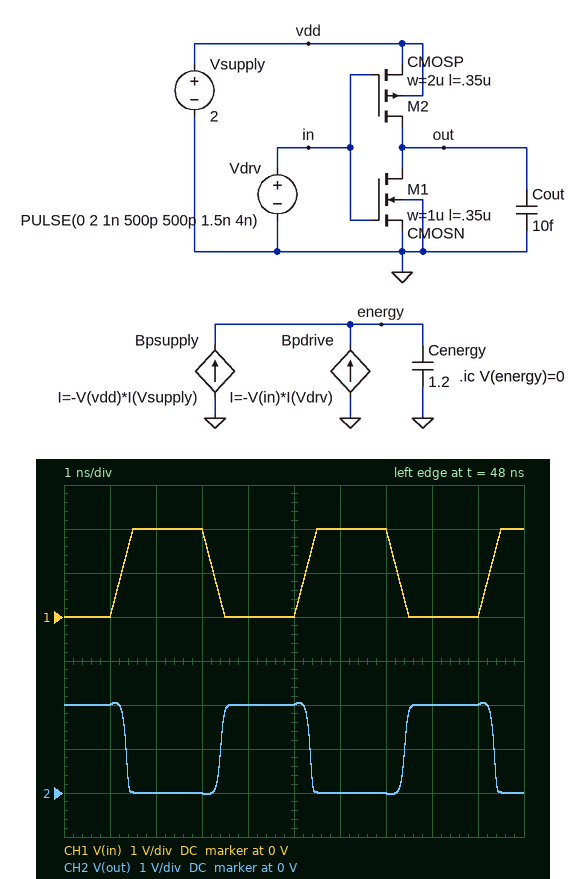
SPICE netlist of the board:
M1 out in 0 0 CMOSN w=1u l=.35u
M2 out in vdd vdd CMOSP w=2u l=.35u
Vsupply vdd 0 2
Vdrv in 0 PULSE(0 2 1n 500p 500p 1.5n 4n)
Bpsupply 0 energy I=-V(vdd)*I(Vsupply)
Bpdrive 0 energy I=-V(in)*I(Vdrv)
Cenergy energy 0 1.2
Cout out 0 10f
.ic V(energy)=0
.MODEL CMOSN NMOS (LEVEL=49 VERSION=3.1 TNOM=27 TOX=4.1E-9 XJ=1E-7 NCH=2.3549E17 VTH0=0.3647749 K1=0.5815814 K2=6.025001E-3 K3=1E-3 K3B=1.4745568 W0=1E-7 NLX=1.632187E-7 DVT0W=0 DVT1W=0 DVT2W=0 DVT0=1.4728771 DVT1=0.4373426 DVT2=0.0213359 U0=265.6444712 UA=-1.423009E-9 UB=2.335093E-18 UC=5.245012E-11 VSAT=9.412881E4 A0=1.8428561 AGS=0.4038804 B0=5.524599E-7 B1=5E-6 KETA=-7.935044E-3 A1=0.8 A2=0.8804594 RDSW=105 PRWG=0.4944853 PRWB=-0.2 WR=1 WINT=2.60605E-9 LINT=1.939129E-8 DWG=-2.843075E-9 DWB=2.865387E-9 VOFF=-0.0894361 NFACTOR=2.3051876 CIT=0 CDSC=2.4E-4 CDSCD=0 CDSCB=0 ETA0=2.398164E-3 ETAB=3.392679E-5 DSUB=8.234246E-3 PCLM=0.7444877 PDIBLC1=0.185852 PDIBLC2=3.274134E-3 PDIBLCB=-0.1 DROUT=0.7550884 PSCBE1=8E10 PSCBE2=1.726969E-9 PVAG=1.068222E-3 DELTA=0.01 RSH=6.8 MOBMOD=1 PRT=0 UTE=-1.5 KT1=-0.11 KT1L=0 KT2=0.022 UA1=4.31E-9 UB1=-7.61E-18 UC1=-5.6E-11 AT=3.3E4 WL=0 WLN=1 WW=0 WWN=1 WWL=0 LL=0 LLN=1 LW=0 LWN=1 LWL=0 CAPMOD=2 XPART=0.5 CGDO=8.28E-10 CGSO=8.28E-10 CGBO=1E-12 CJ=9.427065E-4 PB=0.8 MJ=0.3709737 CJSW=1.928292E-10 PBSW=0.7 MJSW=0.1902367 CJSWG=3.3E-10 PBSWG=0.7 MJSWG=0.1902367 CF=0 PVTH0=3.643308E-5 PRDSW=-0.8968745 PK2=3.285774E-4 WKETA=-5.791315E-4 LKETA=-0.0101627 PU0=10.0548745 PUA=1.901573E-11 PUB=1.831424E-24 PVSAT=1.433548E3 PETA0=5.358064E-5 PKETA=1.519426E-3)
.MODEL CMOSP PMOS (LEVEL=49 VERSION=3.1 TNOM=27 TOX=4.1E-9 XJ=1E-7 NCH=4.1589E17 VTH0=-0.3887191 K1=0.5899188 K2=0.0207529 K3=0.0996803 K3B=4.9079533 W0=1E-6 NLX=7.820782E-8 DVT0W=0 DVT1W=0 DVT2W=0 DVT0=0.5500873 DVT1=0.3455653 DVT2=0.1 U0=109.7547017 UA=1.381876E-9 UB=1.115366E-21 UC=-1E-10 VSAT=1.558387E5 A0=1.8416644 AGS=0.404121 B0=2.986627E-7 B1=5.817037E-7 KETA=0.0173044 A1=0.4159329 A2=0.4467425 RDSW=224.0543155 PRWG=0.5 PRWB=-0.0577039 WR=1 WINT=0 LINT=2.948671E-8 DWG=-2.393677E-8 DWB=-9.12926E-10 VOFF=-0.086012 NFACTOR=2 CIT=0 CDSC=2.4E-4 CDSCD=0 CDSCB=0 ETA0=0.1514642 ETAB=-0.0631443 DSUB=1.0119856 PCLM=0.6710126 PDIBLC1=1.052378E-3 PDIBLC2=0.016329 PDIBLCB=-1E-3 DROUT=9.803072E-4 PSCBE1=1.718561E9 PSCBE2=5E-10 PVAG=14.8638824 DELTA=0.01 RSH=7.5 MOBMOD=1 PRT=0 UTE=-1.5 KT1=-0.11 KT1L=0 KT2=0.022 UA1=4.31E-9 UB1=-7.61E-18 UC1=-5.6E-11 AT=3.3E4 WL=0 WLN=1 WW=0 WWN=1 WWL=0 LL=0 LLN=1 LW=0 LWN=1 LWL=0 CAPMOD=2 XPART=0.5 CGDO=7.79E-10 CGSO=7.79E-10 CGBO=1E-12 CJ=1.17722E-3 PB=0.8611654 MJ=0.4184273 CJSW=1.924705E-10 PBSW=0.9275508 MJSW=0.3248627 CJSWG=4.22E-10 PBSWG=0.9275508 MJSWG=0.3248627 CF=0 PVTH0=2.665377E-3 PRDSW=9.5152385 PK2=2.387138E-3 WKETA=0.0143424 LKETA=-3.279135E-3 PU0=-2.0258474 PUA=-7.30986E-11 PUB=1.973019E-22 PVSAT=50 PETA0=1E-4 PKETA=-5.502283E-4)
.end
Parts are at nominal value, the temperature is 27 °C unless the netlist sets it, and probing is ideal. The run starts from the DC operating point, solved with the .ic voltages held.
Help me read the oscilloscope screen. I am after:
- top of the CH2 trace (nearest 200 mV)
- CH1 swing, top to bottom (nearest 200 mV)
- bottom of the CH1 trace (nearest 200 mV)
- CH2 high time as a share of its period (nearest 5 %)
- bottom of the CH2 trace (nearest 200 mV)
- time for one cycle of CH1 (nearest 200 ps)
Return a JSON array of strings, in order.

["2.0 V", "2.0 V", "0 V", "50 %", "0 V", "4.0 ns"]
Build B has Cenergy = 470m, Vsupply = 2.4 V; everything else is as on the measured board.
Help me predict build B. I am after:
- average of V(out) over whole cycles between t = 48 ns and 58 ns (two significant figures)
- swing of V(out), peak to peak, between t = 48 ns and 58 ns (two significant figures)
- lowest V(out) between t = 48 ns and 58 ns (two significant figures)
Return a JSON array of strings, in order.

["1.2 V", "2.5 V", "-18 mV"]
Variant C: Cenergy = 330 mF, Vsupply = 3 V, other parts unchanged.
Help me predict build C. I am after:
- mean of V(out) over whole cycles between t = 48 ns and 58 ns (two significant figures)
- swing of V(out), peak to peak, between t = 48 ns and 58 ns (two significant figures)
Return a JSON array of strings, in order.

["1.6 V", "3.0 V"]
